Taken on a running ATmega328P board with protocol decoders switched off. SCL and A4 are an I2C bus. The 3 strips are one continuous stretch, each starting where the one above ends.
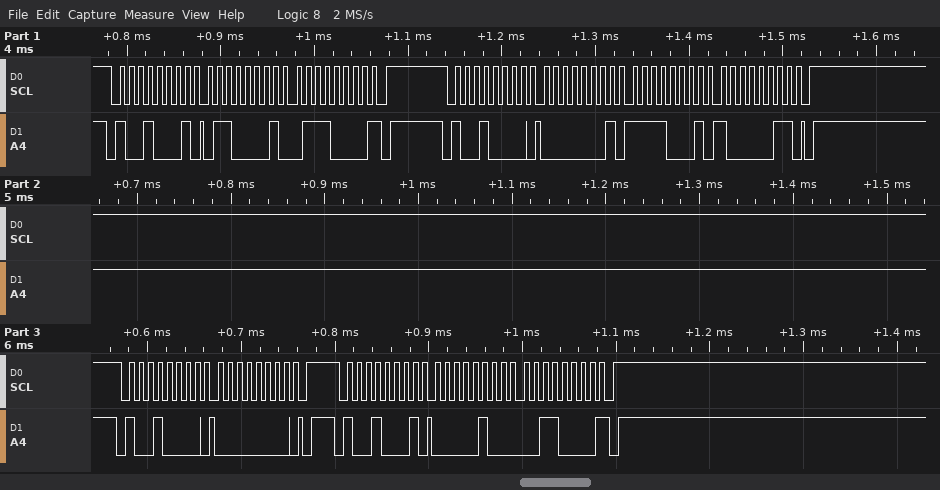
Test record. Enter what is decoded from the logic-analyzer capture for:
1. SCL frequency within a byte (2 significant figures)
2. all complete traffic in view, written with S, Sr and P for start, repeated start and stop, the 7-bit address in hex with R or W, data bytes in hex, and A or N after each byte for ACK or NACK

100 kHz
S 48R A 61 A 70 N P S 48W A 01 A F1 A 83 A P S 48W A 00 A P S 48R A 04 A 30 N P
